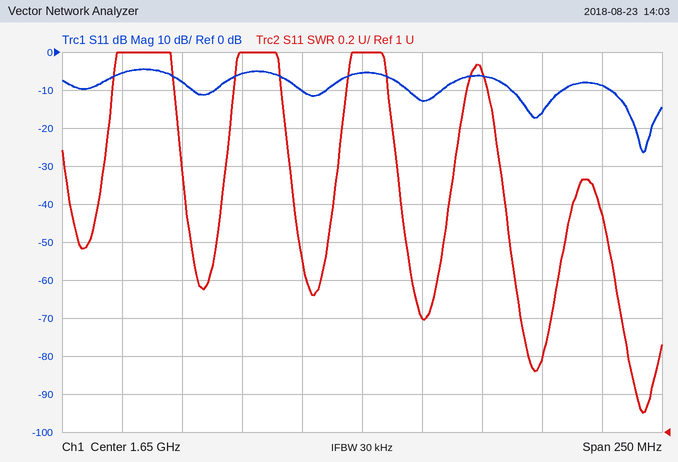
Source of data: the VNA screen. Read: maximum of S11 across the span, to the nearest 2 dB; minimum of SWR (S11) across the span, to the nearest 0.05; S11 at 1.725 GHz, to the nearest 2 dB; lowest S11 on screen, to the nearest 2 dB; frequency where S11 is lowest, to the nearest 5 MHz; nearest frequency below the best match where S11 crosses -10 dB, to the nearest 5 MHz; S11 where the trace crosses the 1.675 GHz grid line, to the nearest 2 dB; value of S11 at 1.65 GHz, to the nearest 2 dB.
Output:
-4 dB
1.10
-16 dB
-26 dB
1.765 GHz
1.755 GHz
-12 dB
-6 dB
